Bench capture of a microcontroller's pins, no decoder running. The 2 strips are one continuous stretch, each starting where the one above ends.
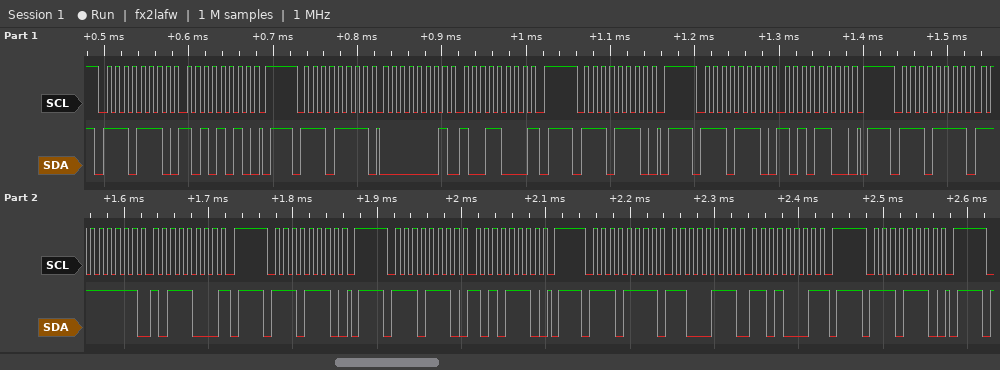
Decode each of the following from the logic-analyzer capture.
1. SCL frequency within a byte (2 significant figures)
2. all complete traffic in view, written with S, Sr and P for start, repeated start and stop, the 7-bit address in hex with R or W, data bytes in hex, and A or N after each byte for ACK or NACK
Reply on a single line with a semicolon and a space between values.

100 kHz; S 77W A AA A P S 77R A 01 A 98 N P S 77W A P S 77W A AC A P S 77R A FF A B8 N P S 77W A P S 77W A AE A P S 77R A C7 A D1 N P S 77W A P
